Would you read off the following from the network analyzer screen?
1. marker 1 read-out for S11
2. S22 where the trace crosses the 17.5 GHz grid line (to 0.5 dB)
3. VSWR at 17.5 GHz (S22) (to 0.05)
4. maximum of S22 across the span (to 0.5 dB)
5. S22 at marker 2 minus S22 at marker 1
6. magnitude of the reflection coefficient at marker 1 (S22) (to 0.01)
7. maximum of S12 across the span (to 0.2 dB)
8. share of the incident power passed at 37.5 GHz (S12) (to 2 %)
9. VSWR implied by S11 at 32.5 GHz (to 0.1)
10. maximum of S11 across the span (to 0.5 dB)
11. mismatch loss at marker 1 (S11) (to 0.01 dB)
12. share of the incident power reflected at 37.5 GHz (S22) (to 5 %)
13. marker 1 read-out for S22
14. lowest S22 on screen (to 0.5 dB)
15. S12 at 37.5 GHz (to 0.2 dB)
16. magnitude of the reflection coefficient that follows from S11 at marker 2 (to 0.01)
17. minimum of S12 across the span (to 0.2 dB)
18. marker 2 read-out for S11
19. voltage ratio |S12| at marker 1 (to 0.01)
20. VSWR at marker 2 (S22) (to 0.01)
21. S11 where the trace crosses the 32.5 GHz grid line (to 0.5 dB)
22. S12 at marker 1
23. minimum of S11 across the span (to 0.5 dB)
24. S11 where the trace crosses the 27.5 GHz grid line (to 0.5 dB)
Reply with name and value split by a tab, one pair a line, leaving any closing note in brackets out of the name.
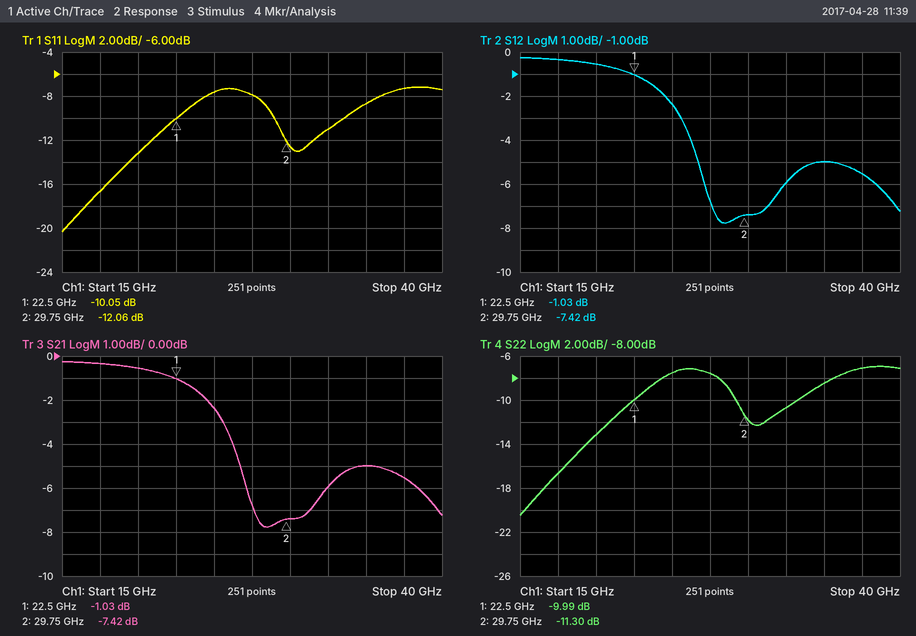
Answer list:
marker 1 read-out for S11	-10.05 dB
S22 where the trace crosses the 17.5 GHz grid line	-16.5 dB
VSWR at 17.5 GHz (S22)	1.35
maximum of S22 across the span	-7.0 dB
S22 at marker 2 minus S22 at marker 1	-1.31 dB
magnitude of the reflection coefficient at marker 1 (S22)	0.32
maximum of S12 across the span	-0.2 dB
share of the incident power passed at 37.5 GHz (S12)	28 %
VSWR implied by S11 at 32.5 GHz	1.8
maximum of S11 across the span	-7.0 dB
mismatch loss at marker 1 (S11)	0.45 dB
share of the incident power reflected at 37.5 GHz (S22)	20 %
marker 1 read-out for S22	-9.99 dB
lowest S22 on screen	-20.5 dB
S12 at 37.5 GHz	-5.6 dB
magnitude of the reflection coefficient that follows from S11 at marker 2	0.25
minimum of S12 across the span	-7.8 dB
marker 2 read-out for S11	-12.06 dB
voltage ratio |S12| at marker 1	0.89
VSWR at marker 2 (S22)	1.75
S11 where the trace crosses the 32.5 GHz grid line	-11.0 dB
S12 at marker 1	-1.03 dB
minimum of S11 across the span	-20.5 dB
S11 where the trace crosses the 27.5 GHz grid line	-8.0 dB
